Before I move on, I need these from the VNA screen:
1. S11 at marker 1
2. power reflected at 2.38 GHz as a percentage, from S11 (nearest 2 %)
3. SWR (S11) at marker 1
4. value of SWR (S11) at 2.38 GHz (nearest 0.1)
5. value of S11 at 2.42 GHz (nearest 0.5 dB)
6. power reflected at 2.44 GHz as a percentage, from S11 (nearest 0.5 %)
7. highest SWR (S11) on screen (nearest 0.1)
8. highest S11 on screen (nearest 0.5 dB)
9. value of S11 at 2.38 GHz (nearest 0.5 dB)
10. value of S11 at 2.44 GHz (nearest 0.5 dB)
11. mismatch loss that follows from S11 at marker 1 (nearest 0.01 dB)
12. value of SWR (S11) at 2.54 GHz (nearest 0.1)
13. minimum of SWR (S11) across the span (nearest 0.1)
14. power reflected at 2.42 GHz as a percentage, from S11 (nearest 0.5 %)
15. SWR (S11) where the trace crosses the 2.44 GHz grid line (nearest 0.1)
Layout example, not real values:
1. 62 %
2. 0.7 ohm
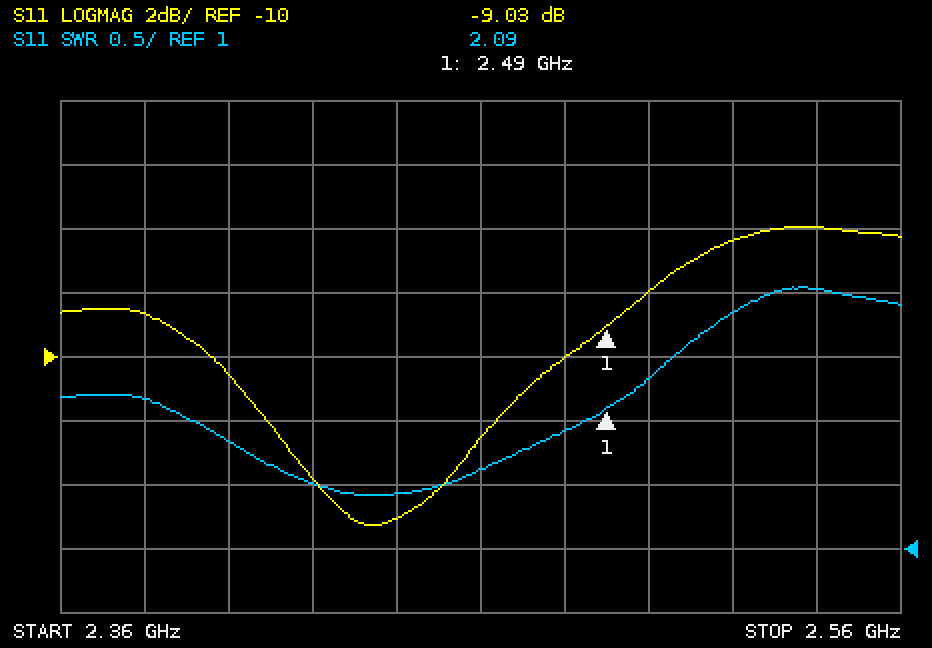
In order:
1. -9.03 dB
2. 14 %
3. 2.09
4. 2.2
5. -14.0 dB
6. 3.0 %
7. 3.0
8. -6.0 dB
9. -8.5 dB
10. -15.0 dB
11. 0.58 dB
12. 3.0
13. 1.4
14. 4.0 %
15. 1.4
